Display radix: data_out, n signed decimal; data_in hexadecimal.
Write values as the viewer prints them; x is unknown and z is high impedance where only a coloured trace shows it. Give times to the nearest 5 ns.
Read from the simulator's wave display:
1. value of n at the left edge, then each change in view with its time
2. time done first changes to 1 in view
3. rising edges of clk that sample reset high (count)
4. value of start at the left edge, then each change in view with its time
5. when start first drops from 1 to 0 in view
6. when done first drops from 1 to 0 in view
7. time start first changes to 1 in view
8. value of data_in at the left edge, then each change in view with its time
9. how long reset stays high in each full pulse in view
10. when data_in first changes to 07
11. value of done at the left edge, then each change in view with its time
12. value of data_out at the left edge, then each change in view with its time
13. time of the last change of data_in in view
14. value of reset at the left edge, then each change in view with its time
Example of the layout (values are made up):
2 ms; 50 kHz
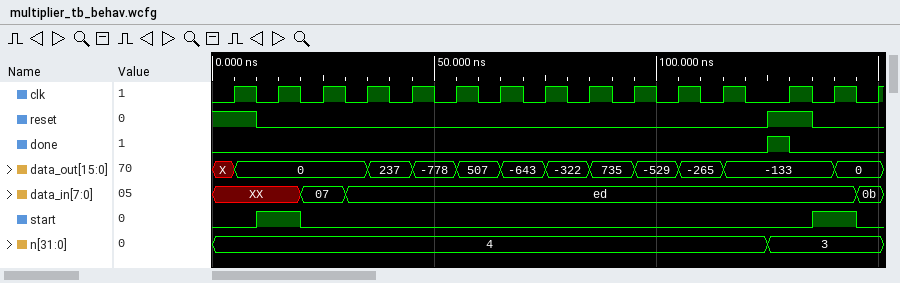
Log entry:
4, 3 at 125 ns; 125 ns; 2; 0, 1 at 10 ns, 0 at 20 ns, 1 at 135 ns, 0 at 145 ns; 20 ns; 130 ns; 10 ns; XX, 07 at 20 ns, ed at 30 ns, 0b at 145 ns; 10 ns; 20 ns; 0, 1 at 125 ns, 0 at 130 ns; X, 0 at 5 ns, 237 at 35 ns, -778 at 45 ns, 507 at 55 ns, -643 at 65 ns, -322 at 75 ns, 735 at 85 ns, -529 at 95 ns, -265 at 105 ns, -133 at 115 ns, 0 at 140 ns; 145 ns; 1, 0 at 10 ns, 1 at 125 ns, 0 at 135 ns
